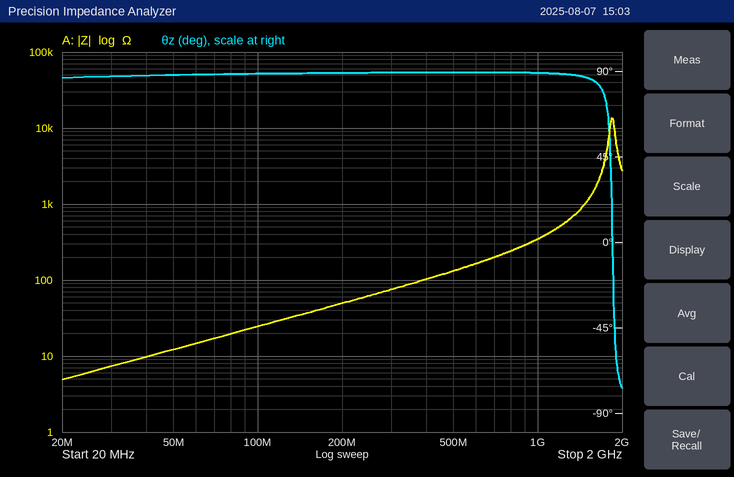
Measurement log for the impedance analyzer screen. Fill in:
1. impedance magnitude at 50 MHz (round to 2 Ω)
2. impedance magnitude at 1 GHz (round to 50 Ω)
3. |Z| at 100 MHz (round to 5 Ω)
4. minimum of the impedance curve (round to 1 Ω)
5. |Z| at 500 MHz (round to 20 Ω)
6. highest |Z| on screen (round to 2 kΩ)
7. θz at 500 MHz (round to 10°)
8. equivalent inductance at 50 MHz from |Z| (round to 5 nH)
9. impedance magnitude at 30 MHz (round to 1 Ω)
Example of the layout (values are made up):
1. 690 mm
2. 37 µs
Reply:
1. 12 Ω
2. 350 Ω
3. 25 Ω
4. 5 Ω
5. 140 Ω
6. 14 kΩ
7. 90°
8. 40 nH
9. 7 Ω
